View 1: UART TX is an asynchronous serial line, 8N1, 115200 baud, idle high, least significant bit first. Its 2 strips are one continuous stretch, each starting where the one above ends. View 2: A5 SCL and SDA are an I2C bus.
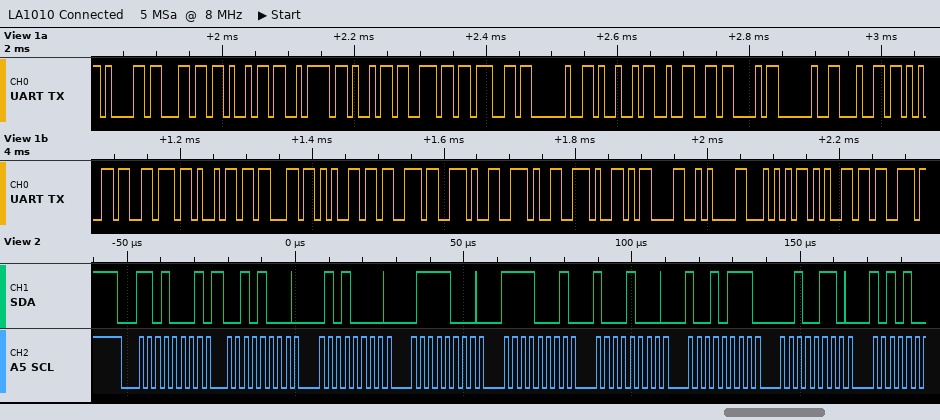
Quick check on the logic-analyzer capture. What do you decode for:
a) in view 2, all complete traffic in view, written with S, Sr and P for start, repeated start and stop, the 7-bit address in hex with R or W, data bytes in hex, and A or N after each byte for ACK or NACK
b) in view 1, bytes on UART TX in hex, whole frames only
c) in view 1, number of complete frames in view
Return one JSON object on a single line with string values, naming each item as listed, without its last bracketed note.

{"in view 2, all complete traffic in view, written with S, Sr and P for start, repeated start and stop, the 7-bit address in hex with R or W, data bytes in hex, and A or N after each byte for ACK or NACK": "S 68R A 28 A 50 A 78 A F1 A 88 A 97 A 26 A", "in view 1, bytes on UART TX in hex, whole frames only": "0x61 0x6C 0x69 0x7A 0x69 0x6E 0x67 0x20 0x49 0x32 0x43 0x20 0x64 0x65 0x76 0x69 0x63 0x65 0x73 0x2E 0x2E 0x2E 0x0D 0x0A 0x54 0x65 0x73", "in view 1, number of complete frames in view": "27"}
